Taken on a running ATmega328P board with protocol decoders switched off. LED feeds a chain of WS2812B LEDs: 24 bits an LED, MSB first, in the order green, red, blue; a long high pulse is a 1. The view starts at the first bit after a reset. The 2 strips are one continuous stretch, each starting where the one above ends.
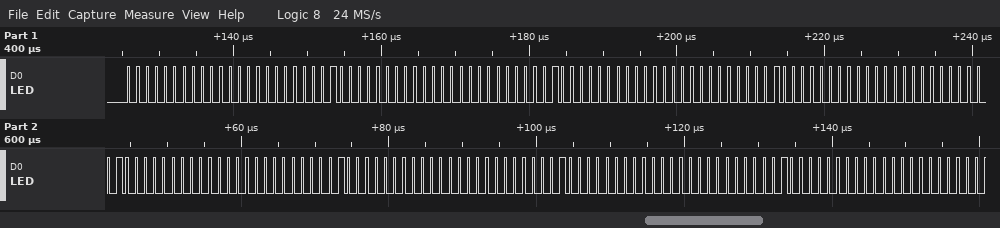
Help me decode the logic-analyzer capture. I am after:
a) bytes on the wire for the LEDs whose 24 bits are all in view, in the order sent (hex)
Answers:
00 00 02 00 00 02 00 00 02 00 00 02 00 00 02 00 00 02 00 00 02
